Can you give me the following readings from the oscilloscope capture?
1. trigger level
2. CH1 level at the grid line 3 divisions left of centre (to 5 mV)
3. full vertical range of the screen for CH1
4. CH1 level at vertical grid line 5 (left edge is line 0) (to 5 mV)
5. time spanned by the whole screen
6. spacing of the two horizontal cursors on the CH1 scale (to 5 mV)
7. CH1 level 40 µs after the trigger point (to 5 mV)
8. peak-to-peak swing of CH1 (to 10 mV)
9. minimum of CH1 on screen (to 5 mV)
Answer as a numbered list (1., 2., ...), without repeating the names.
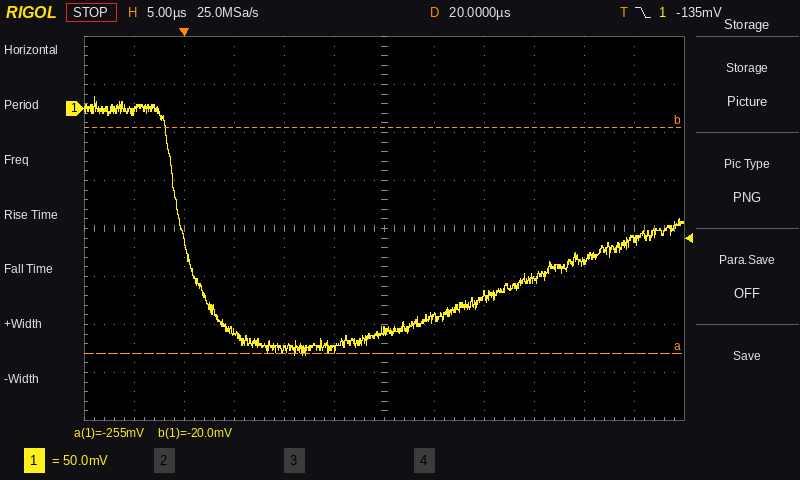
1. -135 mV
2. -230 mV
3. 400 mV
4. -250 mV
5. 60 µs
6. 235 mV
7. -160 mV
8. 270 mV
9. -255 mV
